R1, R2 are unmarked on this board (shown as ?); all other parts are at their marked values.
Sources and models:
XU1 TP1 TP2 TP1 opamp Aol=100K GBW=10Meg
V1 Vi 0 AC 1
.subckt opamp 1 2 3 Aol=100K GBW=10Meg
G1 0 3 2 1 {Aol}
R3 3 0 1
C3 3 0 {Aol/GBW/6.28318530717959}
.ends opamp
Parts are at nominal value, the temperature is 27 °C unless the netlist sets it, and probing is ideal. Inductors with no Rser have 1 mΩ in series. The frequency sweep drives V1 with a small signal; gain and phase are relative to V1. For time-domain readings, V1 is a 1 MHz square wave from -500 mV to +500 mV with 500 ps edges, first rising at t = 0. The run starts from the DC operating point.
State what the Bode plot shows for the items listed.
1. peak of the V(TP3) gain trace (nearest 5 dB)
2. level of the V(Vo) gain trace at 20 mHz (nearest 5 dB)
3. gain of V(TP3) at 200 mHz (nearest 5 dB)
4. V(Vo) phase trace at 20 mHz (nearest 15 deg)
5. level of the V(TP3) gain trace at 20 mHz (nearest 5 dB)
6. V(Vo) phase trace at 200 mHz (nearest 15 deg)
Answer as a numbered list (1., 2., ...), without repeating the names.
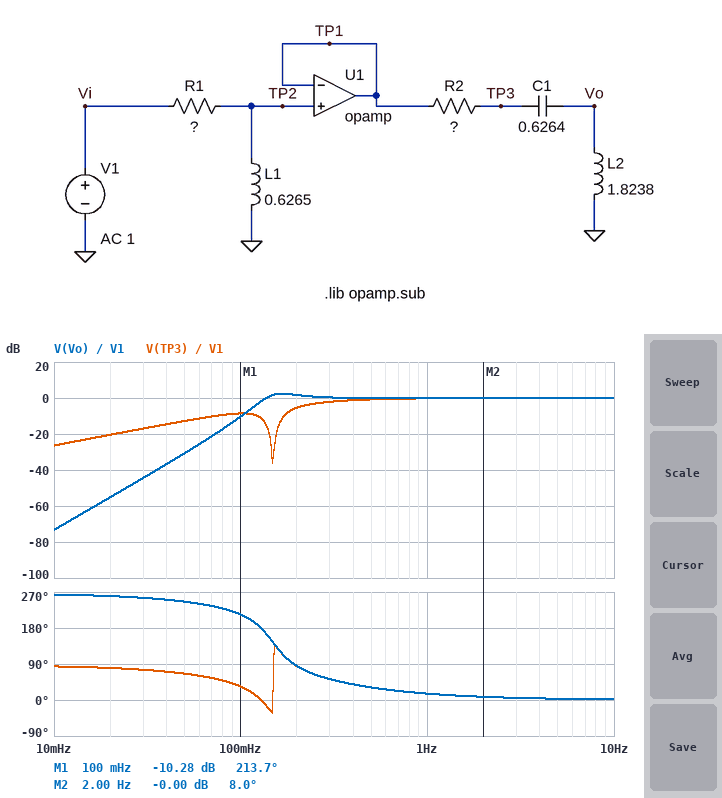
1. 0 dB
2. -55 dB
3. -5 dB
4. 255 deg
5. -20 dB
6. 90 deg
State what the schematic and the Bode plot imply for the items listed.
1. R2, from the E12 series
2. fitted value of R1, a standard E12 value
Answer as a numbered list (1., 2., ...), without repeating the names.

1. 0.82 Ω
2. 0.82 Ω
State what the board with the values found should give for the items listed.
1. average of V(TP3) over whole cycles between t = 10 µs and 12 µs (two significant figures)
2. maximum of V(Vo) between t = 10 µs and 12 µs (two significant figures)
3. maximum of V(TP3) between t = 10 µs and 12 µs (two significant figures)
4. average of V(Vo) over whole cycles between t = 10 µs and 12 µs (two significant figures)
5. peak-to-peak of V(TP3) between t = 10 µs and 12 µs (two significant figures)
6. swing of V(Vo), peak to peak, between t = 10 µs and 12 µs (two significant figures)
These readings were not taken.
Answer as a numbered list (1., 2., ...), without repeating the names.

1. 500 mV
2. 1.0 V
3. 1.0 V
4. 500 mV
5. 1.0 V
6. 1.0 V
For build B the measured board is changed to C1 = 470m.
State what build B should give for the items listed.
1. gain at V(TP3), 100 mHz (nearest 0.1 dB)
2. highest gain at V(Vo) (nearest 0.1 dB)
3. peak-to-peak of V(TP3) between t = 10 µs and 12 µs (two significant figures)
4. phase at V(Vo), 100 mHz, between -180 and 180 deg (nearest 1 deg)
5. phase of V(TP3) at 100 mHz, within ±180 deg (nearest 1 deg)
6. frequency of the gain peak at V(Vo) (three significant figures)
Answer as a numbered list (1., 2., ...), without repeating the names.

1. -7.8 dB
2. 4.2 dB
3. 1.0 V
4. -136 deg
5. 44 deg
6. 186 mHz
